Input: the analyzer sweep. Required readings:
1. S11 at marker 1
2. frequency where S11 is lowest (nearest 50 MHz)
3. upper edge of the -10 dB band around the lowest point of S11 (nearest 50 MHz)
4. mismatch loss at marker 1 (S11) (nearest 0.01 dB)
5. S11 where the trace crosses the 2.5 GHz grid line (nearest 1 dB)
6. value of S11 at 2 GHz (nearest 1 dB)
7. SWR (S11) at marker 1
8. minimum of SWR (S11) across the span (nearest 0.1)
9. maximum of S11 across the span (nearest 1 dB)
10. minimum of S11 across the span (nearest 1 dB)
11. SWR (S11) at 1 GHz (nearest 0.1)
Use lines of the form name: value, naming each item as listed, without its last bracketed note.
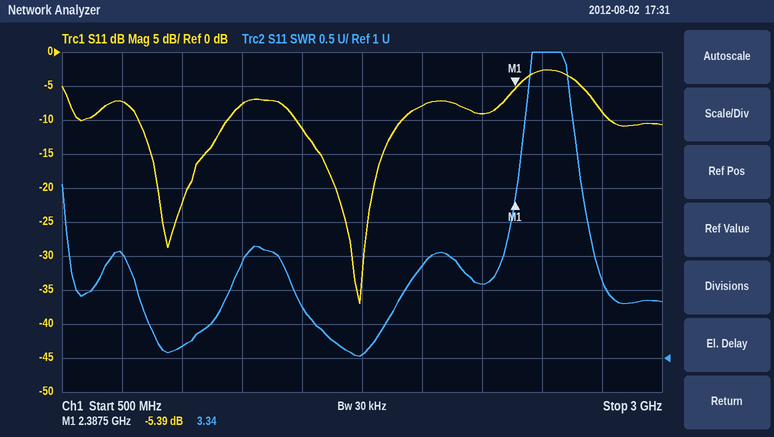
S11 at marker 1: -5.39 dB
frequency where S11 is lowest: 1.75 GHz
upper edge of the -10 dB band around the lowest point of S11: 1.90 GHz
mismatch loss at marker 1 (S11): 1.48 dB
S11 where the trace crosses the 2.5 GHz grid line: -3 dB
value of S11 at 2 GHz: -8 dB
SWR (S11) at marker 1: 3.34
minimum of SWR (S11) across the span: 1.0
maximum of S11 across the span: -3 dB
minimum of S11 across the span: -37 dB
SWR (S11) at 1 GHz: 1.2
